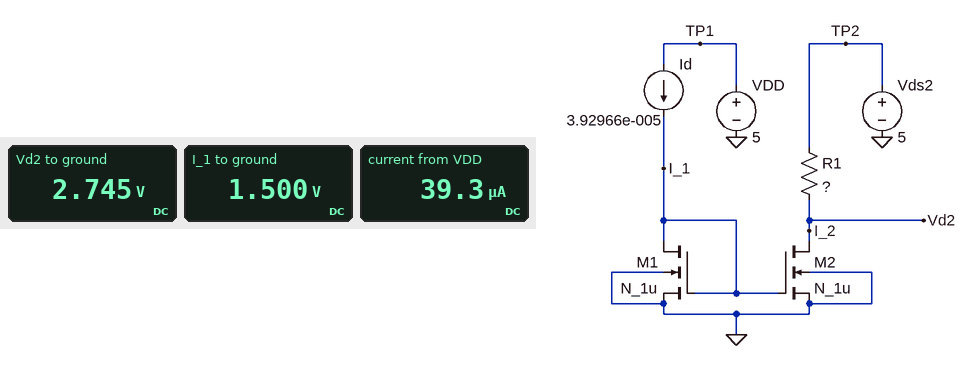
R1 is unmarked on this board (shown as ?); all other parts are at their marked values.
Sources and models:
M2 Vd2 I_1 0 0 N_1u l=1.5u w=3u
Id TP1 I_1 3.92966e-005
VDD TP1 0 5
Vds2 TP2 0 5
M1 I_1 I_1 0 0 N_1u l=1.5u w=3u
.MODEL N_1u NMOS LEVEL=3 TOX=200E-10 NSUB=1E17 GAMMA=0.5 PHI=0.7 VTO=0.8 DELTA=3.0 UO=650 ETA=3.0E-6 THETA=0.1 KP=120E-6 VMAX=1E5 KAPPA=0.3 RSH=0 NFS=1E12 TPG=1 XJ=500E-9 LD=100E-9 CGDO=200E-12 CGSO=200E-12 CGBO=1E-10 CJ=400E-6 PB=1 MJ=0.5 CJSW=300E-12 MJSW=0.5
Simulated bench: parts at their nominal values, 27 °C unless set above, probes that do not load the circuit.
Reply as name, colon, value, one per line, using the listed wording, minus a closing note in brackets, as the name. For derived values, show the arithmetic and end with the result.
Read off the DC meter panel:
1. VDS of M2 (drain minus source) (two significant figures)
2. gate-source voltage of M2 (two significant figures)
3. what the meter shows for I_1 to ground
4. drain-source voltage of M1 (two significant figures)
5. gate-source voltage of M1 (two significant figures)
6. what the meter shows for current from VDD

VDS of M2 (drain minus source): 2.745 V = 2.7 V
gate-source voltage of M2: 1.5 V = 1.5 V
what the meter shows for I_1 to ground: 1.500 V
drain-source voltage of M1: 1.5 V = 1.5 V
gate-source voltage of M1: 1.5 V = 1.5 V
what the meter shows for current from VDD: 39.3 µA
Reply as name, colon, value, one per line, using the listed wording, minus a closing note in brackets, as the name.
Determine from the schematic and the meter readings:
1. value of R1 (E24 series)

value of R1: 56 kΩ
